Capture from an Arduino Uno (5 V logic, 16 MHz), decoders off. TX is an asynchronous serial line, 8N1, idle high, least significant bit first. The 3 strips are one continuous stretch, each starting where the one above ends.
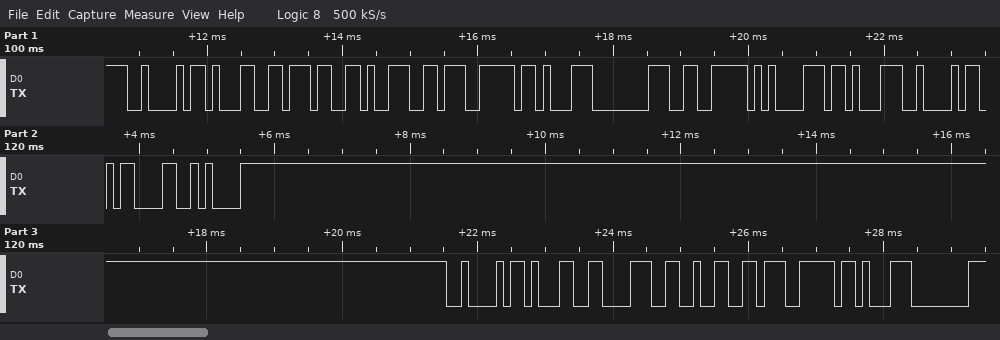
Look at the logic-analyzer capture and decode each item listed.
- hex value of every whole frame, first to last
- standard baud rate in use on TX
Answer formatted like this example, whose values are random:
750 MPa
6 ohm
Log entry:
0x42 0x31 0x37 0x39 0xE7 0x8B 0x80 0xE6 0x85 0x8B 0x42 0x0D 0x0A 0x42 0x31 0x38 0x32 0xE7 0x8B 0x80
9600 baud
